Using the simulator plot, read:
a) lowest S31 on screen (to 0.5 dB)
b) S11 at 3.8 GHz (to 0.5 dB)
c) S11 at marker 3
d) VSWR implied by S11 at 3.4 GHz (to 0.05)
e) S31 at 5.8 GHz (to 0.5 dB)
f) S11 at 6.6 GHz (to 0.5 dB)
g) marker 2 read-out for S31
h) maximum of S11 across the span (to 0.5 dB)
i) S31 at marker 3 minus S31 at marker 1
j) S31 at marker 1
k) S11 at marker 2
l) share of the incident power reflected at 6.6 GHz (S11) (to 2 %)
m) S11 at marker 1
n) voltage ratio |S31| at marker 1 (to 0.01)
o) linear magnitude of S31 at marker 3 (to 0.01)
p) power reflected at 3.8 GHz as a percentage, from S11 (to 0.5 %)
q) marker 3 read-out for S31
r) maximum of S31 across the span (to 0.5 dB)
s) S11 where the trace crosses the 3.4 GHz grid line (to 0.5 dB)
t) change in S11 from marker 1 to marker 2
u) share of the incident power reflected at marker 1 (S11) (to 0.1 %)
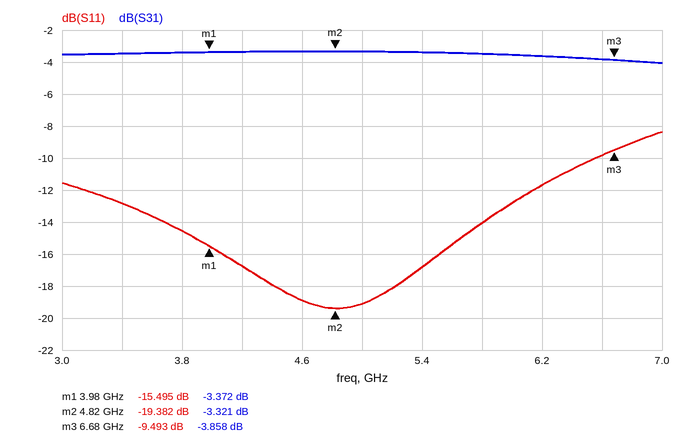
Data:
-4.0 dB
-14.5 dB
-9.493 dB
1.60
-3.5 dB
-10.0 dB
-3.321 dB
-8.5 dB
-0.486 dB
-3.372 dB
-19.382 dB
10 %
-15.495 dB
0.68
0.64
3.5 %
-3.858 dB
-3.5 dB
-13.0 dB
-3.887 dB
2.8 %
